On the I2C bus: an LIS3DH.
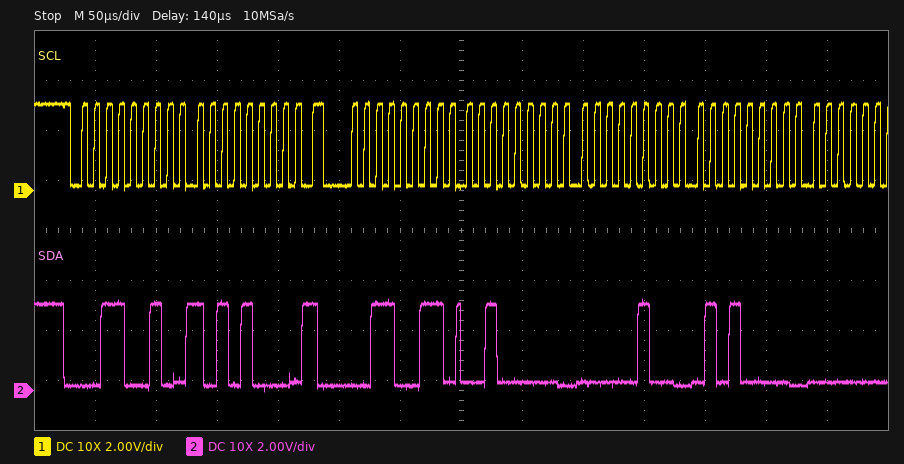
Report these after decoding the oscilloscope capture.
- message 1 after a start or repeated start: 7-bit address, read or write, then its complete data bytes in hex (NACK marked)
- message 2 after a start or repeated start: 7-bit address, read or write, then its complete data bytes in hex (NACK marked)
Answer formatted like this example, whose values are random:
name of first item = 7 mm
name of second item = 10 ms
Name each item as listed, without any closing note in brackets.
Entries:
message 1 after a start or repeated start: 7-bit address, read or write, then its complete data bytes in hex = 0x19 write: A8
message 2 after a start or repeated start: 7-bit address, read or write, then its complete data bytes in hex = 0x19 read: 20 04 50
